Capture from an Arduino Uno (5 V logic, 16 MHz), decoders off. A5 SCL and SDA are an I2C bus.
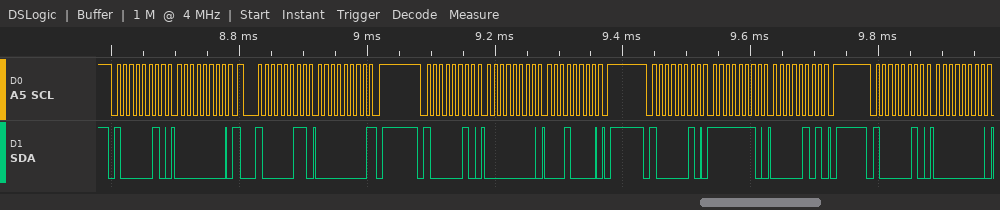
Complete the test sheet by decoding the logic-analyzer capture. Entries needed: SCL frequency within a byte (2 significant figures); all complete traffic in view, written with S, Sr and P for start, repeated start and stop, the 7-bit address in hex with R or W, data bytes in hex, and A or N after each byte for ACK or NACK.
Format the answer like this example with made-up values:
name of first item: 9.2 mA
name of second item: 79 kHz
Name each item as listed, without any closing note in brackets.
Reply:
SCL frequency within a byte: 100 kHz
all complete traffic in view, written with S, Sr and P for start, repeated start and stop, the 7-bit address in hex with R or W, data bytes in hex, and A or N after each byte for ACK or NACK: S 41W A 00 A Sr 41R A 00 N P S 41W A 00 A 10 A P S 41W A FE A 05 A P S 41W A 00 A
